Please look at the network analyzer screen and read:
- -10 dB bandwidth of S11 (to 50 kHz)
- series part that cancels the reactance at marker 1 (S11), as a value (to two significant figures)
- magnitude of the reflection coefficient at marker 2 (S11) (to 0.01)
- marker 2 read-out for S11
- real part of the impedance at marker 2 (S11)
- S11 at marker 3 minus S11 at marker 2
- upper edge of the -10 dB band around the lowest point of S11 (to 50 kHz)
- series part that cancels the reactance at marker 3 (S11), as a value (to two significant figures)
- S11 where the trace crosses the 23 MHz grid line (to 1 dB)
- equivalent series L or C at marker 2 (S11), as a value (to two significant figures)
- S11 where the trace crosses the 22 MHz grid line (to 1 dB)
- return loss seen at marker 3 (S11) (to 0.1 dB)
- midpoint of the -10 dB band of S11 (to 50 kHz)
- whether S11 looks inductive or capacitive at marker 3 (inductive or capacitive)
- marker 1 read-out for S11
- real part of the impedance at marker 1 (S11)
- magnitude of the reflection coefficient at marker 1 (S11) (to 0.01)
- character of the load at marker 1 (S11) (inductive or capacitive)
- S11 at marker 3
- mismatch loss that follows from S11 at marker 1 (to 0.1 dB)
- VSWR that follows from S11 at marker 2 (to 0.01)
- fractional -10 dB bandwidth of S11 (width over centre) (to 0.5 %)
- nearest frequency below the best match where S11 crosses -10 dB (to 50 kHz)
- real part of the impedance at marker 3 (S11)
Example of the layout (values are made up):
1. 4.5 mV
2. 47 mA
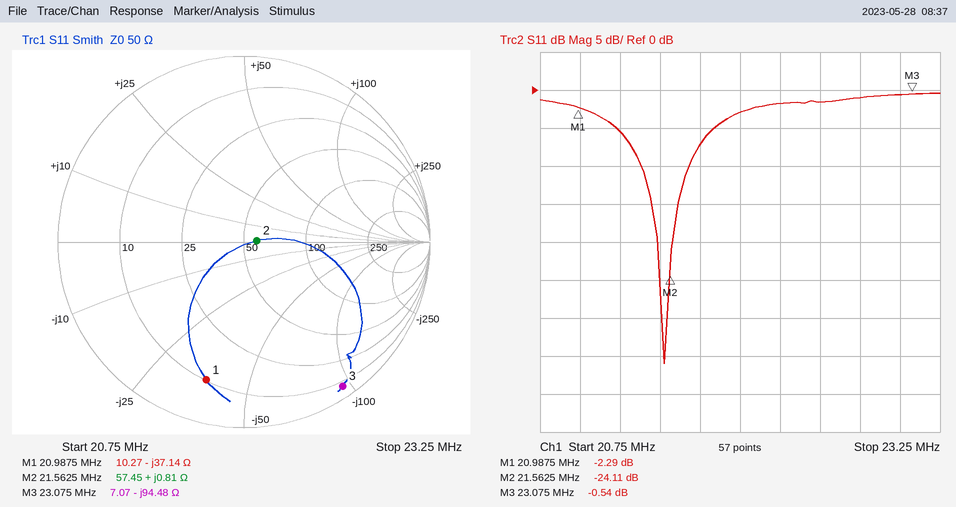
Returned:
1. 300 kHz
2. 280 nH
3. 0.07
4. -24.11 dB
5. 57.45 Ω
6. 23.57 dB
7. 21.70 MHz
8. 650 nH
9. -1 dB
10. 6.0 nH
11. -3 dB
12. 0.5 dB
13. 21.55 MHz
14. capacitive
15. -2.29 dB
16. 10.27 Ω
17. 0.77
18. capacitive
19. -0.54 dB
20. 3.9 dB
21. 1.13
22. 1.5 %
23. 21.40 MHz
24. 7.07 Ω
